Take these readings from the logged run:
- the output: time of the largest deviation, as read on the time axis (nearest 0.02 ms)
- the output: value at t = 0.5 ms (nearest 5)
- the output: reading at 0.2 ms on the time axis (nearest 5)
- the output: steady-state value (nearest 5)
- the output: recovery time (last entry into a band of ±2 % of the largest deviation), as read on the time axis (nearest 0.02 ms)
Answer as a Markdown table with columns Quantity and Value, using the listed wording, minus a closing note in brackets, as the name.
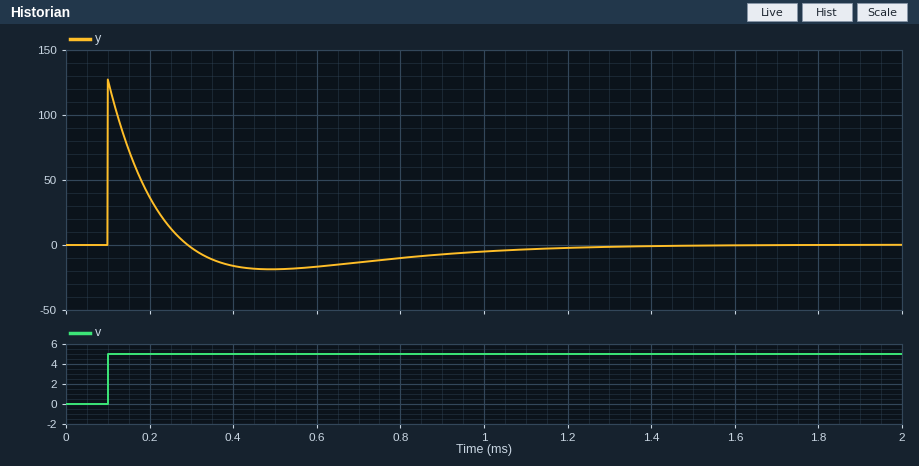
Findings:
| Quantity | Value |
|---|---|
| the output: time of the largest deviation, as read on the time axis | 0.10 ms |
| the output: value at t = 0.5 ms | -20 |
| the output: reading at 0.2 ms on the time axis | 35 |
| the output: steady-state value | 0 |
| the output: recovery time (last entry into a band of ±2 % of the largest deviation), as read on the time axis | 1.18 ms |
